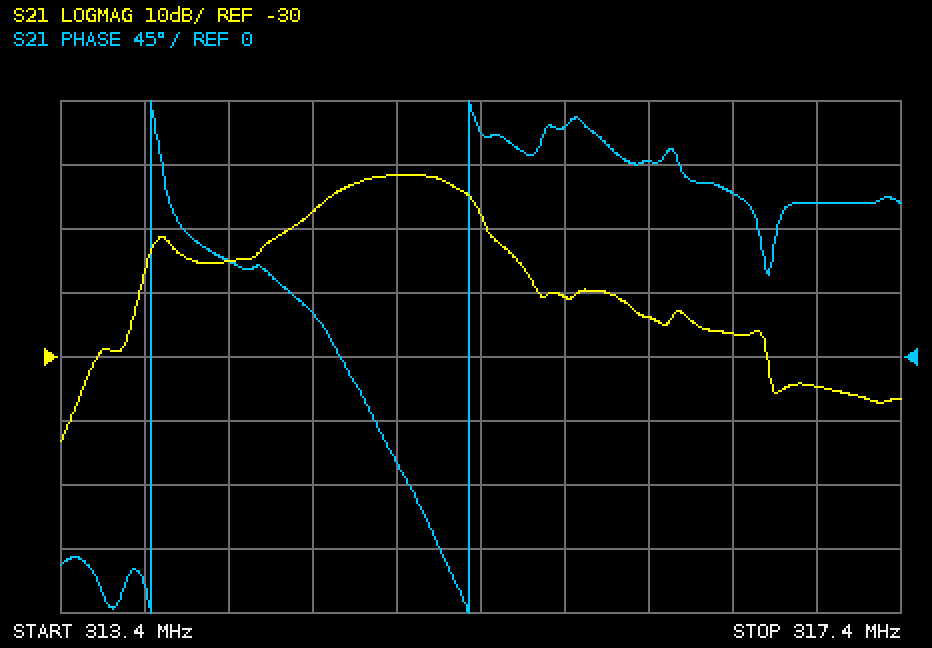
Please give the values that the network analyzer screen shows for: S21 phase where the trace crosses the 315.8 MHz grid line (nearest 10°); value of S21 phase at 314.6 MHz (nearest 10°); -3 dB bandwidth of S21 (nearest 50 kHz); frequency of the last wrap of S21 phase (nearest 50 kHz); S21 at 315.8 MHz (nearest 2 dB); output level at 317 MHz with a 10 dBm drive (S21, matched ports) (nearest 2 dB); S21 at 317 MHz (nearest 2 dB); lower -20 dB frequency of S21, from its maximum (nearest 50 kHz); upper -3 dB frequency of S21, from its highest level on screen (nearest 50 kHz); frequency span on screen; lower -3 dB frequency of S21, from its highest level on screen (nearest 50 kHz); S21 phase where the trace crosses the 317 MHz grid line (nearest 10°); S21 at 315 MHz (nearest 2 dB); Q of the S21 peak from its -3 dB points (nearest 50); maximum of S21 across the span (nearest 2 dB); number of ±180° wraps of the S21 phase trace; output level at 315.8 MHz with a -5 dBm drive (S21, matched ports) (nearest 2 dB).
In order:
160°
30°
650 kHz
315.35 MHz
-20 dB
-24 dBm
-34 dB
313.75 MHz
315.35 MHz
4 MHz
314.70 MHz
110°
-2 dB
500
-2 dB
2
-26 dBm
